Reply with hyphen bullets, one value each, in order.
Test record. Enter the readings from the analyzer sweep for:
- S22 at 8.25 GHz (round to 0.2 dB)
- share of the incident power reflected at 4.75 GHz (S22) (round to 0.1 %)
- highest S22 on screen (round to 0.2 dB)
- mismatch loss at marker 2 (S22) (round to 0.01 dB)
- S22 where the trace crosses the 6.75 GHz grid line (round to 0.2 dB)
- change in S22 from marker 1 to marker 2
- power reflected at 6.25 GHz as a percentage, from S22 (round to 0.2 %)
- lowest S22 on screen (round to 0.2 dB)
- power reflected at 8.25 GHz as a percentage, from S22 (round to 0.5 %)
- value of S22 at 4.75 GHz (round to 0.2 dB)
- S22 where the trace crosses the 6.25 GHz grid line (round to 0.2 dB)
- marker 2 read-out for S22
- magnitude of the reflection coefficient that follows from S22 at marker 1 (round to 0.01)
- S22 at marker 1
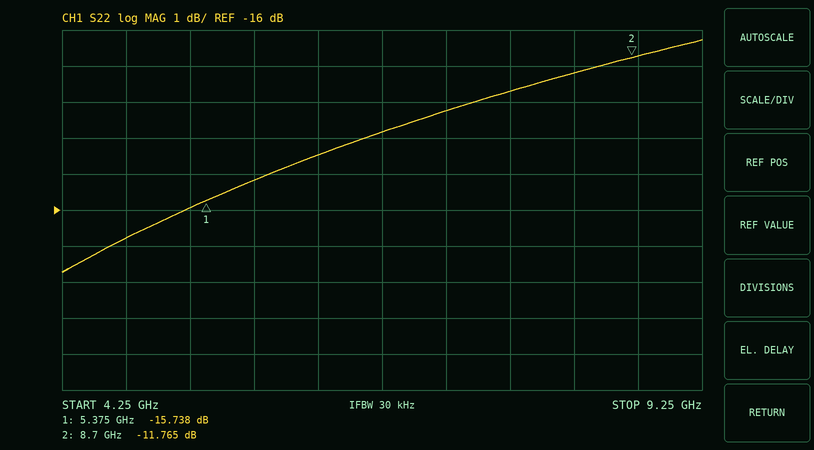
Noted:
- -12.2 dB
- 2.1 %
- -11.2 dB
- 0.30 dB
- -13.8 dB
- 3.973 dB
- 3.6 %
- -17.8 dB
- 6.0 %
- -16.8 dB
- -14.4 dB
- -11.765 dB
- 0.16
- -15.738 dB
